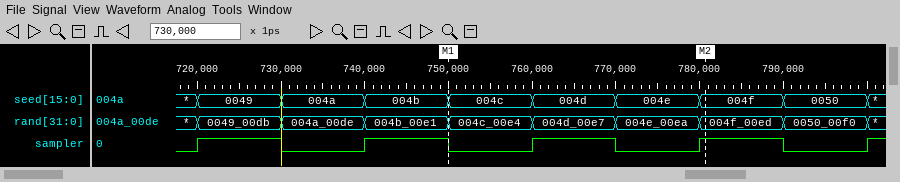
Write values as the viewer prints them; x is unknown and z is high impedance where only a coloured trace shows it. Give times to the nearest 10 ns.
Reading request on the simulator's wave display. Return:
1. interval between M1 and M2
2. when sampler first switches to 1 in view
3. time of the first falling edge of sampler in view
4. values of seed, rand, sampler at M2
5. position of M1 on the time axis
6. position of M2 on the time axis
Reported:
30 ns
720 ns
730 ns
seed=004f, rand=004f_00ed, sampler=1
750 ns
780 ns
